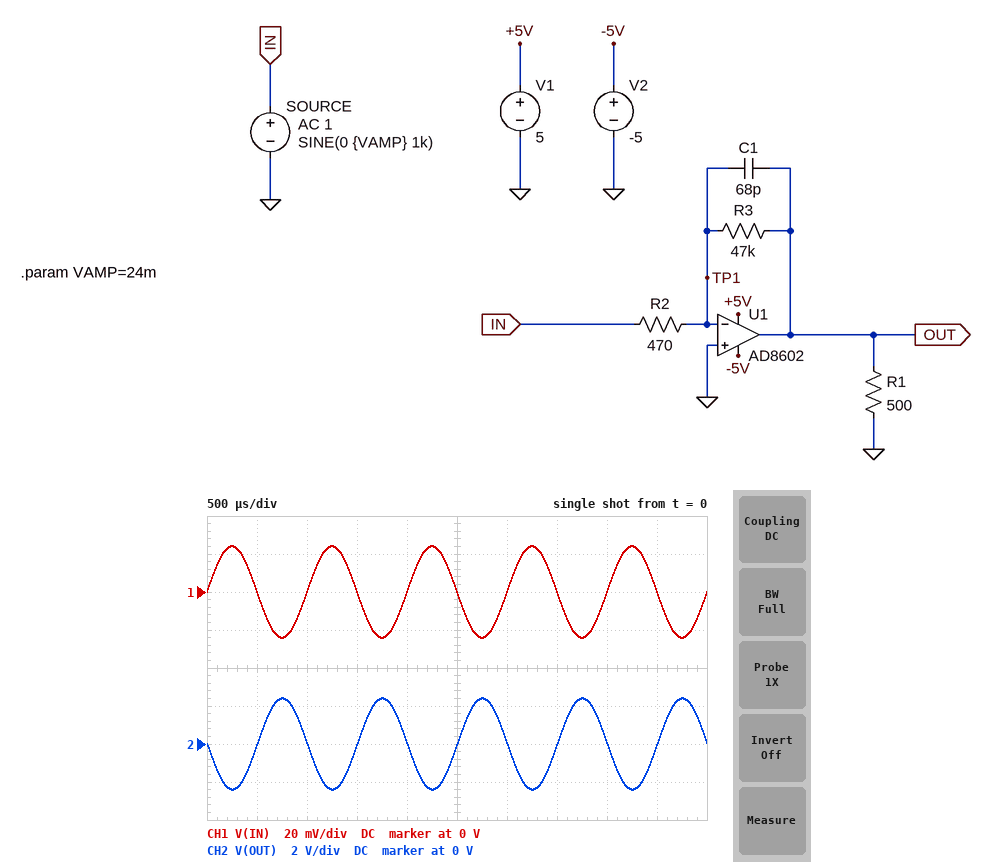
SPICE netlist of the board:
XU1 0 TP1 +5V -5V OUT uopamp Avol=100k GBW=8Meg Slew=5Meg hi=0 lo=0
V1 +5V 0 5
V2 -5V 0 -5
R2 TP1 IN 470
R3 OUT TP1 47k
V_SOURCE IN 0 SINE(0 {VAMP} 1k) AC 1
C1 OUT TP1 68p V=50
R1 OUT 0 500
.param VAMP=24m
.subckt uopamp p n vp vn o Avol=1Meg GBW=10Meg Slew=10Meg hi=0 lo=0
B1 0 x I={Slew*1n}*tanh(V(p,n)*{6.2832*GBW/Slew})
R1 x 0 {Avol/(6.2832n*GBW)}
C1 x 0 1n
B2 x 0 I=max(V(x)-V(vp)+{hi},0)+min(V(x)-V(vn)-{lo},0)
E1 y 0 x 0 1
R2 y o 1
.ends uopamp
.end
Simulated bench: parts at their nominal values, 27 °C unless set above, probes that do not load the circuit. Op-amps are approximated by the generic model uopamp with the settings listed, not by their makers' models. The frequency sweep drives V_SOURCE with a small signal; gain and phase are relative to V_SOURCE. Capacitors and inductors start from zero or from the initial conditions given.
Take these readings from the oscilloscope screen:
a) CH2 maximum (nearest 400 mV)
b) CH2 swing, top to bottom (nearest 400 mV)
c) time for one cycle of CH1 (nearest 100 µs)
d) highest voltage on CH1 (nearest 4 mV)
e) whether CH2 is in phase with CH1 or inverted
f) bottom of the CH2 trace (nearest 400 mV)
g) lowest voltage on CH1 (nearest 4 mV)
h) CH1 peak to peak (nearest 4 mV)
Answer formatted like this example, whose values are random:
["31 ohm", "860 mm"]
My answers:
["2.4 V", "4.8 V", "1.0 ms", "24 mV", "inverted", "-2.4 V", "-24 mV", "48 mV"]
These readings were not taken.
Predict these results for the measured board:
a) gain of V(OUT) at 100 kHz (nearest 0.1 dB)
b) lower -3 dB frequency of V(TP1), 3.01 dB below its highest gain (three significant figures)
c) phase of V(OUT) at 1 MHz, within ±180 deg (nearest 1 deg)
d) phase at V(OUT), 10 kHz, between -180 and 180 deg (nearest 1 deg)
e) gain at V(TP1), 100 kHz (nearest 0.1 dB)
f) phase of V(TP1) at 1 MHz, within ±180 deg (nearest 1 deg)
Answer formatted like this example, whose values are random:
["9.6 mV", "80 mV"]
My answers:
["29.3 dB", "30.5 kHz", "87 deg", "162 deg", "-8.7 dB", "-3 deg"]
